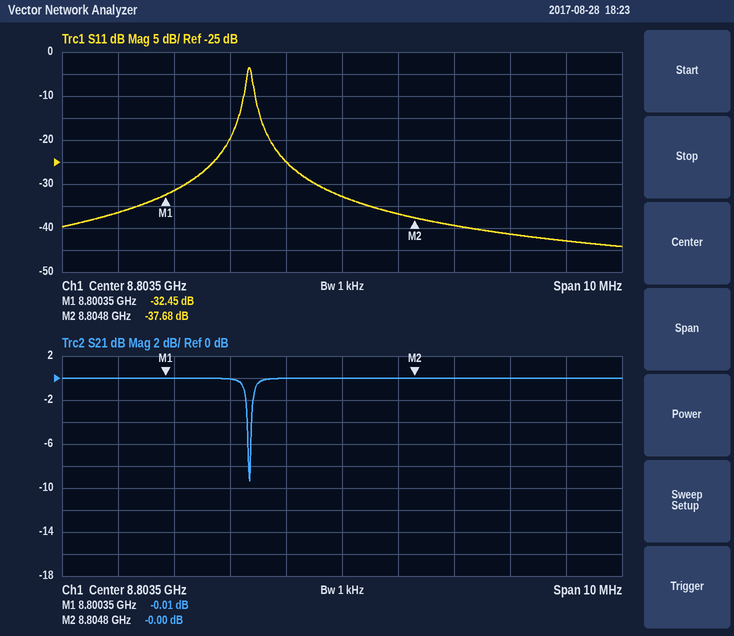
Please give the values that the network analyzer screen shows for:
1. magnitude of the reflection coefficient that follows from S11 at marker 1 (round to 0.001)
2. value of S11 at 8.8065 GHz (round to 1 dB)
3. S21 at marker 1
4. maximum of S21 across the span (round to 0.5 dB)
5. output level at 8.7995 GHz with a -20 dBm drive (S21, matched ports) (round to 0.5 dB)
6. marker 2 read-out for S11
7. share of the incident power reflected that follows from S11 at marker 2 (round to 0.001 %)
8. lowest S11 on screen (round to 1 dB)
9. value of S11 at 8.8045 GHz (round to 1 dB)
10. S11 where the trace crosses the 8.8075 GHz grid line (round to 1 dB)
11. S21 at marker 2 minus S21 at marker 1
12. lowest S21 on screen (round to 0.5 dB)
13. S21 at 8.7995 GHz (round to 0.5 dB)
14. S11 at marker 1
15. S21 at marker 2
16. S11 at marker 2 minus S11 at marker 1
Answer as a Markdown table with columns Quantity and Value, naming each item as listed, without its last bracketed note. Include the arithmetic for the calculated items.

| Quantity | Value |
|---|---|
| magnitude of the reflection coefficient that follows from S11 at marker 1 | 10^(-32.45/20) ≈ 0.024 |
| value of S11 at 8.8065 GHz | -41 dB |
| S21 at marker 1 | -0.01 dB |
| maximum of S21 across the span | 0.0 dB |
| output level at 8.7995 GHz with a -20 dBm drive (S21, matched ports) | -20 dBm + (0.0 dB) = -20.0 dBm |
| marker 2 read-out for S11 | -37.68 dB |
| share of the incident power reflected that follows from S11 at marker 2 | 10^(-37.68/10) ≈ 0.017 % |
| lowest S11 on screen | -44 dB |
| value of S11 at 8.8045 GHz | -37 dB |
| S11 where the trace crosses the 8.8075 GHz grid line | -43 dB |
| S21 at marker 2 minus S21 at marker 1 | -0 − (-0.01) = 0.01 dB |
| lowest S21 on screen | -9.5 dB |
| S21 at 8.7995 GHz | 0.0 dB |
| S11 at marker 1 | -32.45 dB |
| S21 at marker 2 | -0.00 dB |
| S11 at marker 2 minus S11 at marker 1 | -37.68 − (-32.45) = -5.23 dB |
